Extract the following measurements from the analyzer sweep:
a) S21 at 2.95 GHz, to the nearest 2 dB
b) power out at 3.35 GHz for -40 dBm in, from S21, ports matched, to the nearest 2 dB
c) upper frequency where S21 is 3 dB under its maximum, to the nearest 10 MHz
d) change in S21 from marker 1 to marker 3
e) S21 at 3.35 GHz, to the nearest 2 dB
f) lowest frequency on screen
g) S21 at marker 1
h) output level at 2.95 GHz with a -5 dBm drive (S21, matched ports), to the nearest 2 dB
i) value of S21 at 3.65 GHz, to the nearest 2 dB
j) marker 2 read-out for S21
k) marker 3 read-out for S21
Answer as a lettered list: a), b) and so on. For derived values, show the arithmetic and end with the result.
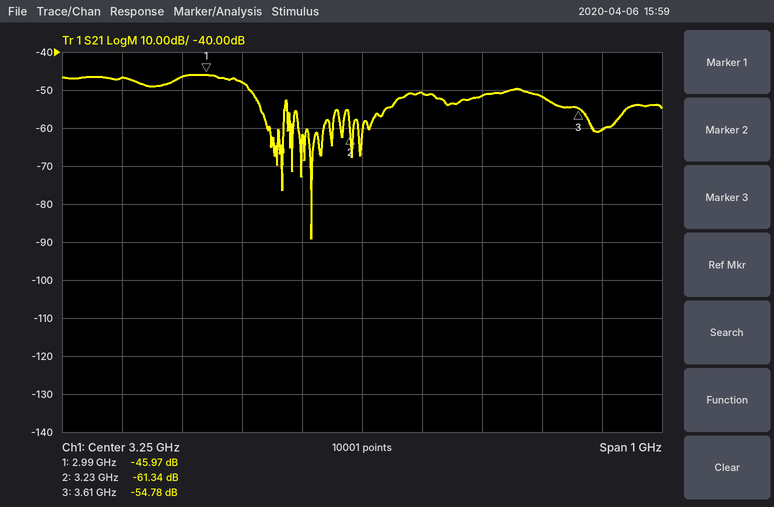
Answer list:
a) -46 dB
b) -40 dBm + (-50 dB) = -90 dBm
c) 3.06 GHz
d) -54.78 − (-45.97) = -8.81 dB
e) -50 dB
f) 2.75 GHz
g) -45.97 dB
h) -5 dBm + (-46 dB) = -52 dBm
i) -60 dB
j) -61.34 dB
k) -54.78 dB
